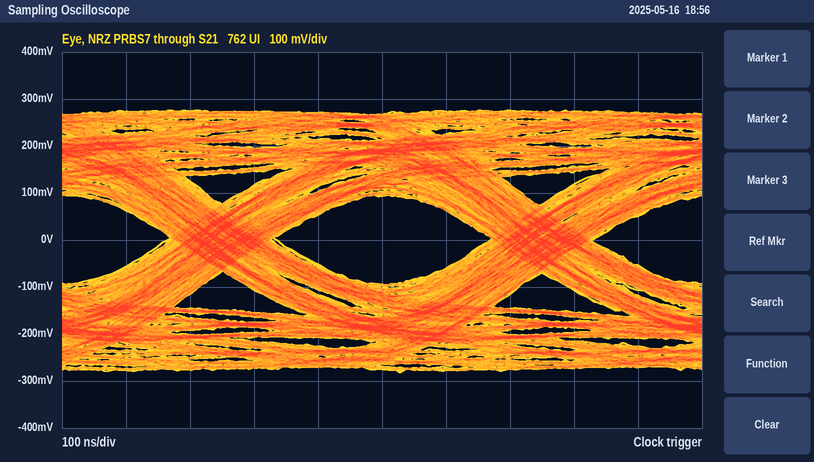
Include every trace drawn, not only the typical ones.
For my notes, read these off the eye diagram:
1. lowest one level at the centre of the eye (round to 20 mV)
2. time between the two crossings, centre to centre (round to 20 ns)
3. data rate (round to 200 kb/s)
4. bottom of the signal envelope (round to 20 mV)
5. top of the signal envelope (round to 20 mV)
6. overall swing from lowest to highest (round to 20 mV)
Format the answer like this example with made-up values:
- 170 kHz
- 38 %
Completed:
- 100 mV
- 500 ns
- 2.0 Mb/s
- -280 mV
- 280 mV
- 560 mV
